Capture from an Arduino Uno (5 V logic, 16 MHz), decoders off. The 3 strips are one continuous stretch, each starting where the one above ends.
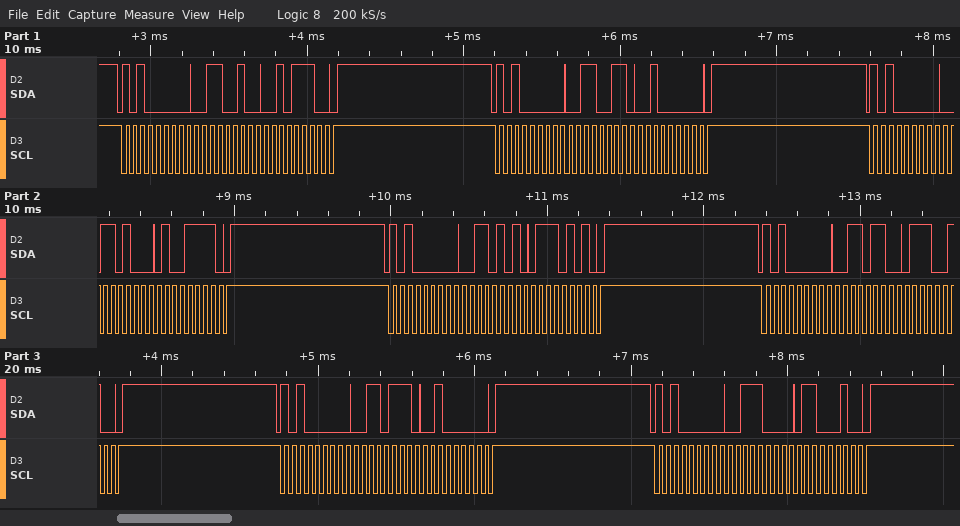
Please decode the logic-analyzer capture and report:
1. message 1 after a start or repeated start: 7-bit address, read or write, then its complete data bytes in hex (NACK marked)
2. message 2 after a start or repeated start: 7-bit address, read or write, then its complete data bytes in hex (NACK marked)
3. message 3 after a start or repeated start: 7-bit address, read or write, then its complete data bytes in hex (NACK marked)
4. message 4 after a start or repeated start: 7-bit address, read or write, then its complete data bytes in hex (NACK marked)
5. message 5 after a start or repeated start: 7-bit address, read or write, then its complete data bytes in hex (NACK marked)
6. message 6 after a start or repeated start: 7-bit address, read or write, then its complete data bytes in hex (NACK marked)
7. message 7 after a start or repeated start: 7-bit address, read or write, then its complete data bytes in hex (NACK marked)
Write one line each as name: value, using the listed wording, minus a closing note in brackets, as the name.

message 1 after a start or repeated start: 7-bit address, read or write, then its complete data bytes in hex: 0x50 write: 32 2E
message 2 after a start or repeated start: 7-bit address, read or write, then its complete data bytes in hex: 0x50 write: 33 20
message 3 after a start or repeated start: 7-bit address, read or write, then its complete data bytes in hex: 0x50 write: 34 4F
message 4 after a start or repeated start: 7-bit address, read or write, then its complete data bytes in hex: 0x50 write: 35 75
message 5 after a start or repeated start: 7-bit address, read or write, then its complete data bytes in hex: 0x50 write: 36 72
message 6 after a start or repeated start: 7-bit address, read or write, then its complete data bytes in hex: 0x50 write: 37 20
message 7 after a start or repeated start: 7-bit address, read or write, then its complete data bytes in hex: 0x50 write: 38 62
